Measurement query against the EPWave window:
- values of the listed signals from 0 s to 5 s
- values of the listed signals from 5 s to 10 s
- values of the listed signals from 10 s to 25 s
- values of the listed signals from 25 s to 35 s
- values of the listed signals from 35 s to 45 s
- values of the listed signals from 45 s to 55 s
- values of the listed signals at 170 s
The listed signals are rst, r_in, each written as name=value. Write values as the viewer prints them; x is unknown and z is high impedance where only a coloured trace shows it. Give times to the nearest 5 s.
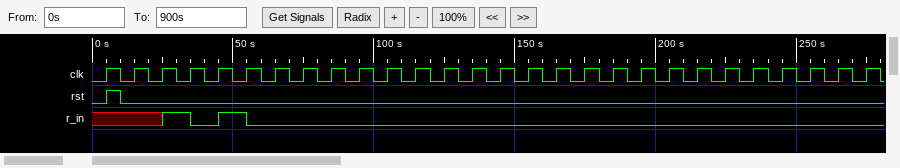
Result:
rst=0, r_in=x
rst=1, r_in=x
rst=0, r_in=x
rst=0, r_in=1
rst=0, r_in=0
rst=0, r_in=1
rst=0, r_in=0
